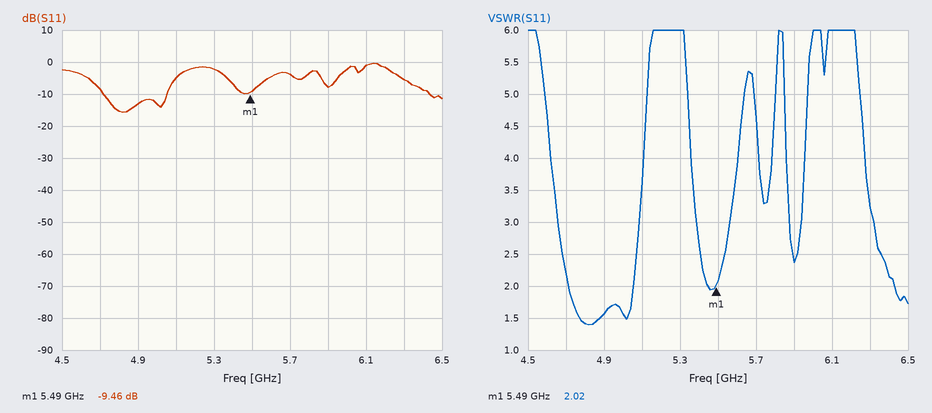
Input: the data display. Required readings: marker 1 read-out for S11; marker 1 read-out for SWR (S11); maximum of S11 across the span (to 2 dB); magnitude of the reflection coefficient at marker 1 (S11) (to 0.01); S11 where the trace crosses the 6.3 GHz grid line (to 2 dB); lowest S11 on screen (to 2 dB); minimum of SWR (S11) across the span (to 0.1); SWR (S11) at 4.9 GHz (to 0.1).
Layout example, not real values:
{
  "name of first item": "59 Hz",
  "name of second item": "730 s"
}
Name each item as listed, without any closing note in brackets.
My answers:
{
  "marker 1 read-out for S11": "-9.46 dB",
  "marker 1 read-out for SWR": "2.02",
  "maximum of S11 across the span": "0 dB",
  "magnitude of the reflection coefficient at marker 1 (S11)": "0.34",
  "S11 where the trace crosses the 6.3 GHz grid line": "-6 dB",
  "lowest S11 on screen": "-16 dB",
  "minimum of SWR (S11) across the span": "1.4",
  "SWR (S11) at 4.9 GHz": "1.6"
}
